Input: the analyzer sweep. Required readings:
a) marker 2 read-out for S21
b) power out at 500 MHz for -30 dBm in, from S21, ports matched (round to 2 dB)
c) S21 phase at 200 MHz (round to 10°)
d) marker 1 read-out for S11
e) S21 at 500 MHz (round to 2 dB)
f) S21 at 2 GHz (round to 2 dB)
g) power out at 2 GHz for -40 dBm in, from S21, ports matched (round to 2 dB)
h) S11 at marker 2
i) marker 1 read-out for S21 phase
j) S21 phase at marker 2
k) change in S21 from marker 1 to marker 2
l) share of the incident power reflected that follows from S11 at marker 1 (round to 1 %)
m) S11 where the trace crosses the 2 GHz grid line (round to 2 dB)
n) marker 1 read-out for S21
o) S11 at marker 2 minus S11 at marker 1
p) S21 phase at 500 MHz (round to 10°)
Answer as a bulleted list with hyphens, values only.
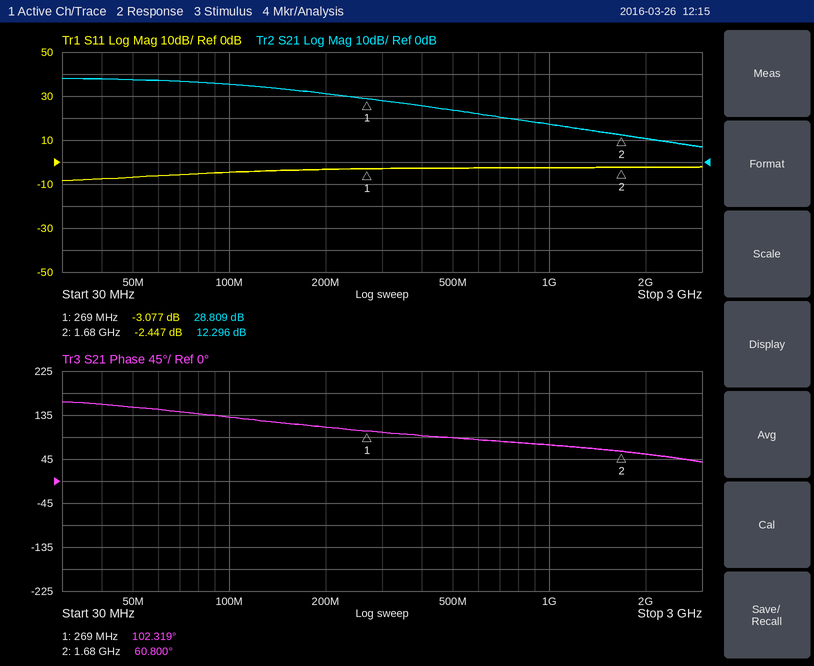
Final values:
- 12.296 dB
- -6 dBm
- 110°
- -3.077 dB
- 24 dB
- 10 dB
- -30 dBm
- -2.447 dB
- 102.319°
- 60.800°
- -16.513 dB
- 49 %
- -2 dB
- 28.809 dB
- 0.630 dB
- 90°
